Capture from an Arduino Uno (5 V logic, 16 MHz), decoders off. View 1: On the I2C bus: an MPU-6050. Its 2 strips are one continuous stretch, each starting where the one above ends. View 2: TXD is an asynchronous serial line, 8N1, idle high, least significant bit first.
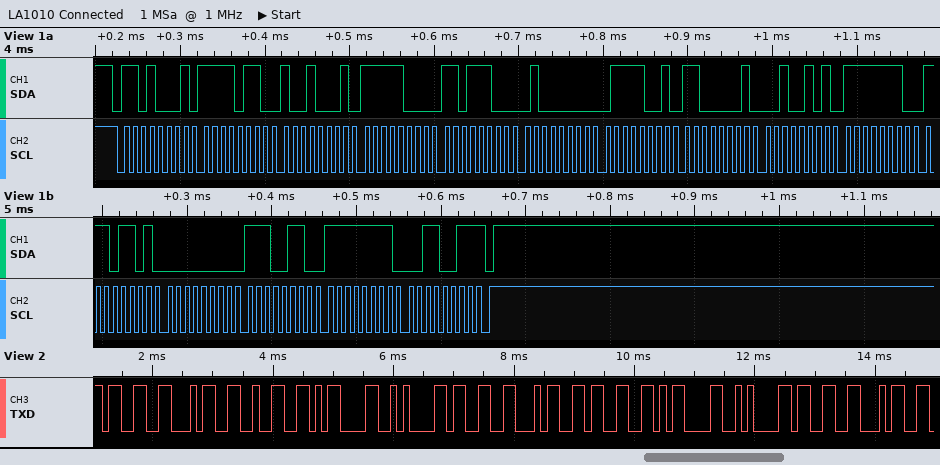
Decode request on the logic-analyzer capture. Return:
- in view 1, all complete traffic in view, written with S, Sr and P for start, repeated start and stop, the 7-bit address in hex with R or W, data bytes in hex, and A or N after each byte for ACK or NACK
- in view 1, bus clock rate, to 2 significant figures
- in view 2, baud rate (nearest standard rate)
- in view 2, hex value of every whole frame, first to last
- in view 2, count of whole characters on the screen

S 68R A F6 A 91 A F8 A DC A 40 A 79 A C1 A 25 A FE A ED A 00 A E6 A FF A 33 N P
100 kHz
9600 baud
0x33 0x34 0x32 0x0D 0x0A 0x33 0x34 0x33 0x0D 0x0A 0x33 0x34
12
